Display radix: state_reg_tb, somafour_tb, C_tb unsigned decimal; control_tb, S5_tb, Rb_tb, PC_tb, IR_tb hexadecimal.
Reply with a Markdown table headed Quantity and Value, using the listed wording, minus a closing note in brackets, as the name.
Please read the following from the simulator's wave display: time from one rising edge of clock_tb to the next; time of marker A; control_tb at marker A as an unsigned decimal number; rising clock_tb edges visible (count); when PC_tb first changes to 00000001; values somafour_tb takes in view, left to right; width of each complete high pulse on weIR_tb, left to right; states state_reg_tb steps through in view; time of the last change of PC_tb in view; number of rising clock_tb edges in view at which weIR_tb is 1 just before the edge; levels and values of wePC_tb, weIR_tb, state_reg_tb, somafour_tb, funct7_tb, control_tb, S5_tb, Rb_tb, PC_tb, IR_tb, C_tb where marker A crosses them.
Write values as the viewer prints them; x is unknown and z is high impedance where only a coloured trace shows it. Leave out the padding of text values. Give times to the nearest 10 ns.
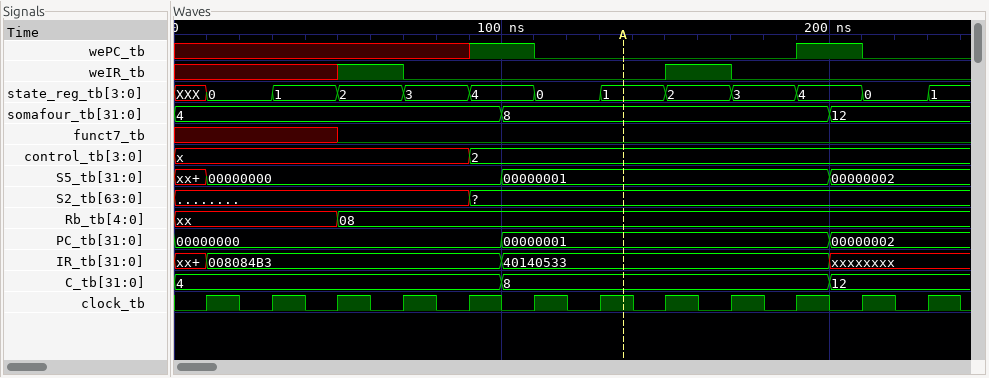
| Quantity | Value |
|---|---|
| time from one rising edge of clock_tb to the next | 20 ns |
| time of marker A | 140 ns |
| control_tb at marker A as an unsigned decimal number | 2 |
| rising clock_tb edges visible | 12 |
| when PC_tb first changes to 00000001 | 100 ns |
| values somafour_tb takes in view, left to right | 4, 8, 12 |
| width of each complete high pulse on weIR_tb, left to right | 20 ns |
| states state_reg_tb steps through in view | XXX, 0, 1, 2, 3, 4, 0, 1, 2, 3, 4, 0, 1 |
| time of the last change of PC_tb in view | 200 ns |
| number of rising clock_tb edges in view at which weIR_tb is 1 just before the edge | 2 |
| levels and values of wePC_tb, weIR_tb, state_reg_tb, somafour_tb, funct7_tb, control_tb, S5_tb, Rb_tb, PC_tb, IR_tb, C_tb where marker A crosses them | wePC_tb=0, weIR_tb=0, state_reg_tb=1, somafour_tb=8, funct7_tb=0, control_tb=2, S5_tb=00000001, Rb_tb=08, PC_tb=00000001, IR_tb=40140533, C_tb=8 |
